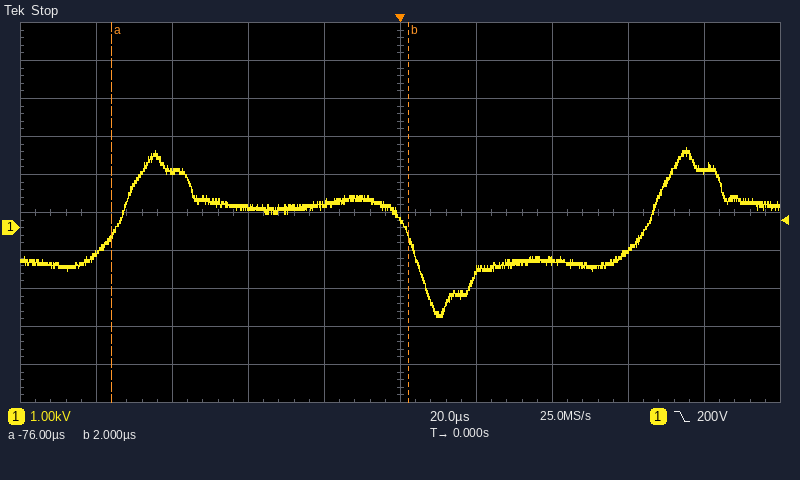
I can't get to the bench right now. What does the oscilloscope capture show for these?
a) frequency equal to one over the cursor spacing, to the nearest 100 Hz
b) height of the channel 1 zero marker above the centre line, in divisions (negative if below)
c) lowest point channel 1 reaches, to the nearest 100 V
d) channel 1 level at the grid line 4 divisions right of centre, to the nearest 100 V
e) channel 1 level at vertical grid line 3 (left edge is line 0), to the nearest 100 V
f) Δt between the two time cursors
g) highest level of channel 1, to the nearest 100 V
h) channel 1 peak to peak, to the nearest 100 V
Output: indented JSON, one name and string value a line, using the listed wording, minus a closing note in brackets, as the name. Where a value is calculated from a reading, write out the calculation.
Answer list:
{
  "frequency equal to one over the cursor spacing, to the nearest 100 Hz": "1 / 78 µs ≈ 12.8 kHz",
  "height of the channel 1 zero marker above the centre line, in divisions": "-0.4 div",
  "lowest point channel 1 reaches, to the nearest 100 V": "-2.4 kV",
  "channel 1 level at the grid line 4 divisions right of centre, to the nearest 100 V": "1.5 kV",
  "channel 1 level at vertical grid line 3 (left edge is line 0), to the nearest 100 V": "500 V",
  "Δt between the two time cursors": "2 µs − (-76 µs) = 78 µs",
  "highest level of channel 1, to the nearest 100 V": "2.1 kV",
  "channel 1 peak to peak, to the nearest 100 V": "2.1 kV − (-2.4 kV) = 4.5 kV"
}
